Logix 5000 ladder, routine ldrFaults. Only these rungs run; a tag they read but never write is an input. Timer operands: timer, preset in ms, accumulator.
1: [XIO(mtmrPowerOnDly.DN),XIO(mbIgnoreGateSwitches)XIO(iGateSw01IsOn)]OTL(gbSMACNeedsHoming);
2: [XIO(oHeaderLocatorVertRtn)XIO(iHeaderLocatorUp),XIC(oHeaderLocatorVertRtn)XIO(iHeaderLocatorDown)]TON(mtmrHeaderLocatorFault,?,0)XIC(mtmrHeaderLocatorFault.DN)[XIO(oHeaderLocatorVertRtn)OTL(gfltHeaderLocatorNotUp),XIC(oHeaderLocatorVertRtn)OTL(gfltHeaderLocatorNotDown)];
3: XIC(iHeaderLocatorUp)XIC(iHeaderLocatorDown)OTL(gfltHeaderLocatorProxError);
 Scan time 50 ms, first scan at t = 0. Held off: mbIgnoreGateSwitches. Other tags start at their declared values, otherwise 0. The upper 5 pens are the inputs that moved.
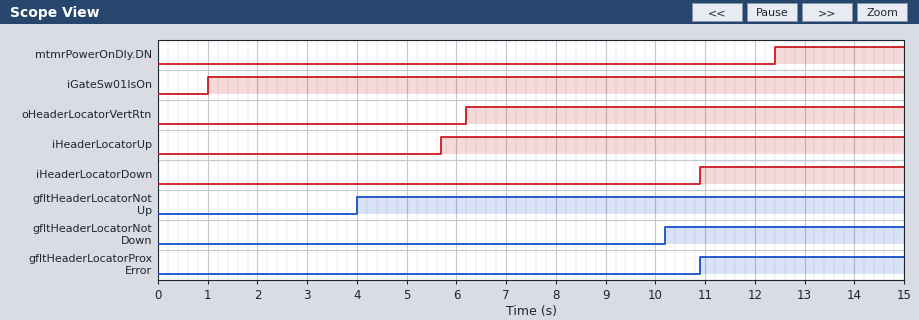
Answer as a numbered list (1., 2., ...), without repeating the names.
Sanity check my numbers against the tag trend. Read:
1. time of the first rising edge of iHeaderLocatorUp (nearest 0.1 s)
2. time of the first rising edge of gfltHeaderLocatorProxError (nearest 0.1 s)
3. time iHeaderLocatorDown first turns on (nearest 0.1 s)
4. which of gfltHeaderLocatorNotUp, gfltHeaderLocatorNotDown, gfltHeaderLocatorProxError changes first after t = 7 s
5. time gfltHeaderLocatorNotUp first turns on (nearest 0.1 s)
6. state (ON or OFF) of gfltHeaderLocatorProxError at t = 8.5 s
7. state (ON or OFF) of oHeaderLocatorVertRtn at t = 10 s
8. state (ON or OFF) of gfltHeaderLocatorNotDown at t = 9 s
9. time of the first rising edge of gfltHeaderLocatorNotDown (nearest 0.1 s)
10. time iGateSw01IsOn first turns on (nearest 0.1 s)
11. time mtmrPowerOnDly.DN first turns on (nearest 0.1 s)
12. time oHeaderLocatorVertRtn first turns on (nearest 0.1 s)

1. 5.7 s
2. 10.9 s
3. 10.9 s
4. gfltHeaderLocatorNotDown
5. 4.0 s
6. OFF
7. ON
8. OFF
9. 10.2 s
10. 1.0 s
11. 12.4 s
12. 6.2 s
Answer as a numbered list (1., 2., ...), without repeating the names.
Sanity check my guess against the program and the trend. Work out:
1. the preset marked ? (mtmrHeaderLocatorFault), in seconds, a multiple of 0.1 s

1. 4.0 s
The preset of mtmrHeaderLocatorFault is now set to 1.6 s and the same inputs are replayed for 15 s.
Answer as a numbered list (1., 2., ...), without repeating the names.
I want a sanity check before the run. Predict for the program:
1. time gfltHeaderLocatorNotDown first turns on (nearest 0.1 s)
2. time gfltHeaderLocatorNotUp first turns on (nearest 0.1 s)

1. 7.8 s
2. 1.6 s
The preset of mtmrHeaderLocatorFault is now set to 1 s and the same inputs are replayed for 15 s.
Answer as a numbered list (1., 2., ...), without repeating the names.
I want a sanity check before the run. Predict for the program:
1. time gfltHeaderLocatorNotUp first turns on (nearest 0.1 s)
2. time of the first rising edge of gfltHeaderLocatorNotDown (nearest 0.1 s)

1. 1.0 s
2. 7.2 s
